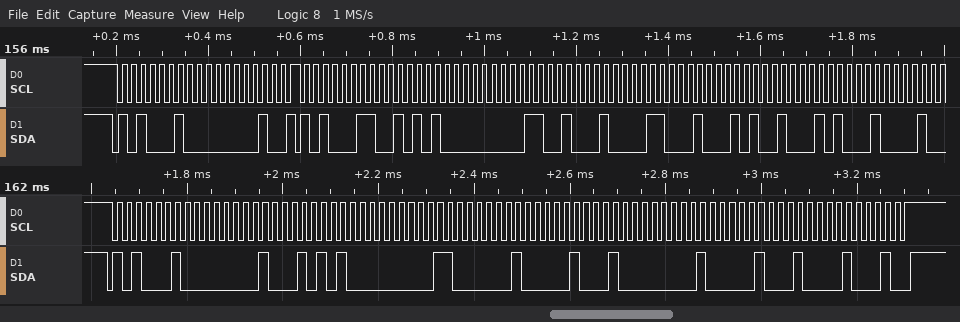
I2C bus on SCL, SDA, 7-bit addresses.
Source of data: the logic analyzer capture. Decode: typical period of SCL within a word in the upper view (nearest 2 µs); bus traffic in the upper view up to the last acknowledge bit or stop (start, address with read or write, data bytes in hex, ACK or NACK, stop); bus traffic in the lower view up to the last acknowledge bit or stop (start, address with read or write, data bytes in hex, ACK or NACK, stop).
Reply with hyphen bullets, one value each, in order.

- 20 µs
- start, address 51 write ACK, 02 ACK, repeated start, address 51 read ACK, 54 ACK, 03 ACK, 44 ACK, 62 ACK, 52 ACK, 51 ACK
- start, address 51 write ACK, 02 ACK, 54 ACK, 03 ACK, 04 ACK, 22 ACK, 02 ACK, 11 ACK, 11 ACK, stop
